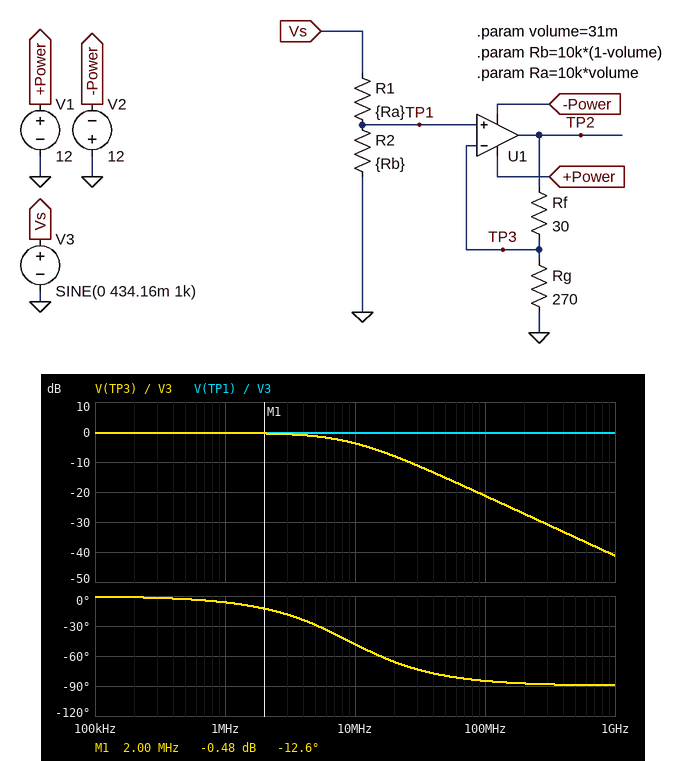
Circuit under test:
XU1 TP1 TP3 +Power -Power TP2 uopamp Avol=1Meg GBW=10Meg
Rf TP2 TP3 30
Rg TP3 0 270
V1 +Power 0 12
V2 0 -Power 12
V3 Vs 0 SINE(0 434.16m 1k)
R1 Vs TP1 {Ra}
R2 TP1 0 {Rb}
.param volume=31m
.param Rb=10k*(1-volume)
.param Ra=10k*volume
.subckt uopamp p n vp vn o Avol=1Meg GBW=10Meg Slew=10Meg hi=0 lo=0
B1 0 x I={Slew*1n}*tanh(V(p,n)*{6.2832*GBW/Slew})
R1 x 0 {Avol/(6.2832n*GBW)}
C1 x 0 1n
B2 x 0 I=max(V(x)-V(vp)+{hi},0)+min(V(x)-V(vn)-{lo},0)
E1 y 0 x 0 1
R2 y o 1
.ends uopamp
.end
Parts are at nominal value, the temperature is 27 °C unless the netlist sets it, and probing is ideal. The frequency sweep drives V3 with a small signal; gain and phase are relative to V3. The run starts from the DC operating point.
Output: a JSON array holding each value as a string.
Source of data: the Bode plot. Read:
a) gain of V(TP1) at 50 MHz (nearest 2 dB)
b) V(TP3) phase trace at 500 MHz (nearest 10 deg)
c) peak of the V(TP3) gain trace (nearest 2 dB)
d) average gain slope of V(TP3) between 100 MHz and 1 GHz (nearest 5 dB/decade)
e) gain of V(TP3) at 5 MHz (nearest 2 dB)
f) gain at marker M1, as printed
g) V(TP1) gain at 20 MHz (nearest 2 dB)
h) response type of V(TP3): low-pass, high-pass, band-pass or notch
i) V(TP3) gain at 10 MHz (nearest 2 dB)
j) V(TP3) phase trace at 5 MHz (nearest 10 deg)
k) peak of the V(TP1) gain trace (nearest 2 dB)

["0 dB", "-90 deg", "0 dB", "-20 dB/decade", "-2 dB", "-0.48 dB", "0 dB", "low-pass", "-4 dB", "-30 deg", "0 dB"]
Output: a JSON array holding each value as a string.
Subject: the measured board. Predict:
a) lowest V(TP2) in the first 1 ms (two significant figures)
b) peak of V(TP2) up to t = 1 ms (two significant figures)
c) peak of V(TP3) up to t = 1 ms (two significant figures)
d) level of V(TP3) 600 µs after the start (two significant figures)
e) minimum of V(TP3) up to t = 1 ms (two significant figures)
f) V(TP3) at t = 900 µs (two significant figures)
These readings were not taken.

["-470 mV", "470 mV", "420 mV", "-250 mV", "-420 mV", "-250 mV"]
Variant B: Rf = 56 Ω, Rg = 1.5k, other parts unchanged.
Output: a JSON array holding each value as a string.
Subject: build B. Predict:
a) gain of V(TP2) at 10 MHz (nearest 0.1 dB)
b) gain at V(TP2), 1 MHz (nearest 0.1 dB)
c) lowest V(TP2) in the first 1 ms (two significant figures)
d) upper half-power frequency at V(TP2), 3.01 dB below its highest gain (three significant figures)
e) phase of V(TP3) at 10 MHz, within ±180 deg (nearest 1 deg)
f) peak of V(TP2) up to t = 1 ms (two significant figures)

["-3.1 dB", "0 dB", "-440 mV", "9.63 MHz", "-46 deg", "440 mV"]
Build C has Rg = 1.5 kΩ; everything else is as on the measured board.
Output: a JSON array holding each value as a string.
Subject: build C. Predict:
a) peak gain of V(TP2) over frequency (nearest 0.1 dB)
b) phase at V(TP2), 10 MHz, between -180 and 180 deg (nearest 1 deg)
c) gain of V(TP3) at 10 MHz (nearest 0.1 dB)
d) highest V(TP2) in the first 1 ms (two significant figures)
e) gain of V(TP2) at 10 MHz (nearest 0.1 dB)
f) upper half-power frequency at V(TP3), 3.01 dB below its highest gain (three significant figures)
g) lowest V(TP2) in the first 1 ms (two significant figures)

["-0.1 dB", "-46 deg", "-3.4 dB", "430 mV", "-3.2 dB", "9.80 MHz", "-430 mV"]
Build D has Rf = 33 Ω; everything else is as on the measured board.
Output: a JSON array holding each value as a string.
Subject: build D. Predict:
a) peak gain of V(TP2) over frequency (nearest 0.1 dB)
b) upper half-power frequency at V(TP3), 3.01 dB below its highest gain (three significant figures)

["0.7 dB", "8.88 MHz"]
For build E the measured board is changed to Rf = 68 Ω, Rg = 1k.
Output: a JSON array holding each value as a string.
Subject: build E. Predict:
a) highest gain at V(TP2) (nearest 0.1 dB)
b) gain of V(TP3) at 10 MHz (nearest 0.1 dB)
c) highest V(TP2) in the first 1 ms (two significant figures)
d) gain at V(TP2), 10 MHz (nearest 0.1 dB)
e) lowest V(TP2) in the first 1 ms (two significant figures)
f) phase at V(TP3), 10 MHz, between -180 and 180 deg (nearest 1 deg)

["0.3 dB", "-3.6 dB", "450 mV", "-3.0 dB", "-450 mV", "-47 deg"]
